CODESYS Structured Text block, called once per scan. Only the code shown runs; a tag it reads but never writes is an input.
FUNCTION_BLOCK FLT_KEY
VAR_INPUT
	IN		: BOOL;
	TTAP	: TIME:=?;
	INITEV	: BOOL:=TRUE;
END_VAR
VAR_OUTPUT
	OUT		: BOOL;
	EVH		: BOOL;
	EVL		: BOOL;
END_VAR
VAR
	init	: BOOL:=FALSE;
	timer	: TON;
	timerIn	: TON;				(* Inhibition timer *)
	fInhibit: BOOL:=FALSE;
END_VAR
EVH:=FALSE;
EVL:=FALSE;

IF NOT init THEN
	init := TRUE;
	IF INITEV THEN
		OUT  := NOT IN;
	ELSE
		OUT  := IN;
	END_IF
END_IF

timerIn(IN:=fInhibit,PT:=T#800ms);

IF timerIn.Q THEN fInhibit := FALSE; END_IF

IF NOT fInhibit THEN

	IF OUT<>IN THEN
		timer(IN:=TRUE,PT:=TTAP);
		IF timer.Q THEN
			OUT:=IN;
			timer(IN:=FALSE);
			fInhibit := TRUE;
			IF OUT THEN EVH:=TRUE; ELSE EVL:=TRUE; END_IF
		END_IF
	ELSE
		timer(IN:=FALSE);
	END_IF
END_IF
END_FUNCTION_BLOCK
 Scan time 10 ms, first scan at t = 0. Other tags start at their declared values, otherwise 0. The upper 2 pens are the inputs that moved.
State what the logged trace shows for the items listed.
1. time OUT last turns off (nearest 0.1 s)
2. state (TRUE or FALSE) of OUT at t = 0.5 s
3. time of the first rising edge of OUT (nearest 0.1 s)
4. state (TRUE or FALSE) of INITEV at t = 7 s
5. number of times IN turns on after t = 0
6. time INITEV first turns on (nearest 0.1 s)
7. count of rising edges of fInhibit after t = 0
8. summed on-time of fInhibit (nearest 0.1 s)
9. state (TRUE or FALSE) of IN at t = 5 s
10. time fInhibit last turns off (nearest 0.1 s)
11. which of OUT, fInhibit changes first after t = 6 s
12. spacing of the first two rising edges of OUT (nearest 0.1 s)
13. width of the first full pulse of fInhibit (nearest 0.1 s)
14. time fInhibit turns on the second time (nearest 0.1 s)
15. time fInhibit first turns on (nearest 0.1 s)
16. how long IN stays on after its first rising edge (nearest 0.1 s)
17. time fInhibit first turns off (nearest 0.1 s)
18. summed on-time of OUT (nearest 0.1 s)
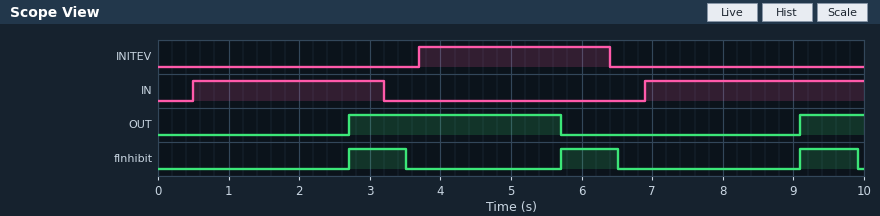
5.7 s
FALSE
2.7 s
FALSE
2
3.7 s
3
2.4 s
FALSE
9.9 s
fInhibit
6.4 s
0.8 s
5.7 s
2.7 s
2.7 s
3.5 s
3.9 s
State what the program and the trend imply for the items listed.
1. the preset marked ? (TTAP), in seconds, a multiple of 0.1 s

2.2 s
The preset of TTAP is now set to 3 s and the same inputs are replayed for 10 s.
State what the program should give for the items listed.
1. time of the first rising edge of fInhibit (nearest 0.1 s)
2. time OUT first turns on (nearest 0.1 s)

9.9 s
9.9 s
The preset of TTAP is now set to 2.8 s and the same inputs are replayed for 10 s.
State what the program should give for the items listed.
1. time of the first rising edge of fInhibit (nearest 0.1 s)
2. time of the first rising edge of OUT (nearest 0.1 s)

9.7 s
9.7 s
